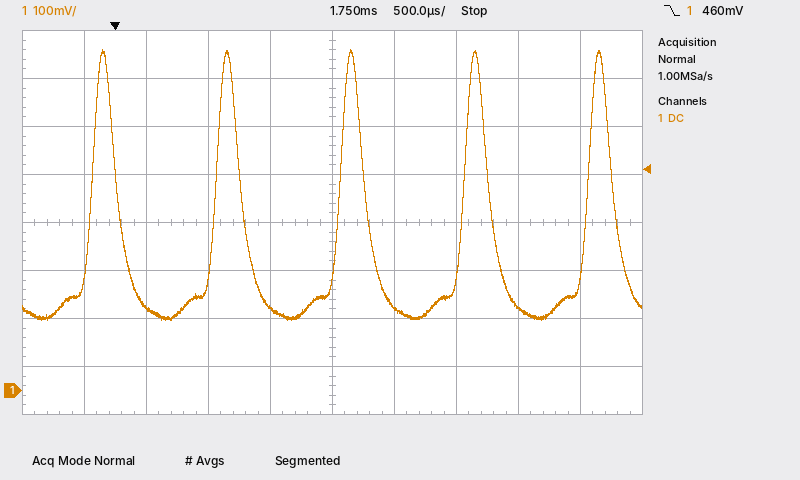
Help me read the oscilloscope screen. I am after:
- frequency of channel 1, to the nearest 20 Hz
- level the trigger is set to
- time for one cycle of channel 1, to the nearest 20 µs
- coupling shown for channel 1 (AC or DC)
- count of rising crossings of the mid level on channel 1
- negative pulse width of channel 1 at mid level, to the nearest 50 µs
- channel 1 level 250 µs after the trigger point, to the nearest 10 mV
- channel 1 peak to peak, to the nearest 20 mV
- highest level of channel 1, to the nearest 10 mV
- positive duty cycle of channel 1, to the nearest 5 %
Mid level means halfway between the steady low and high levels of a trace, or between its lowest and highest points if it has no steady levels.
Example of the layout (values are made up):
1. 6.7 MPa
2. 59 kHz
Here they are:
1. 1.00 kHz
2. 460 mV
3. 1.00 ms
4. DC
5. 5
6. 800 µs
7. 170 mV
8. 560 mV
9. 710 mV
10. 20 %
